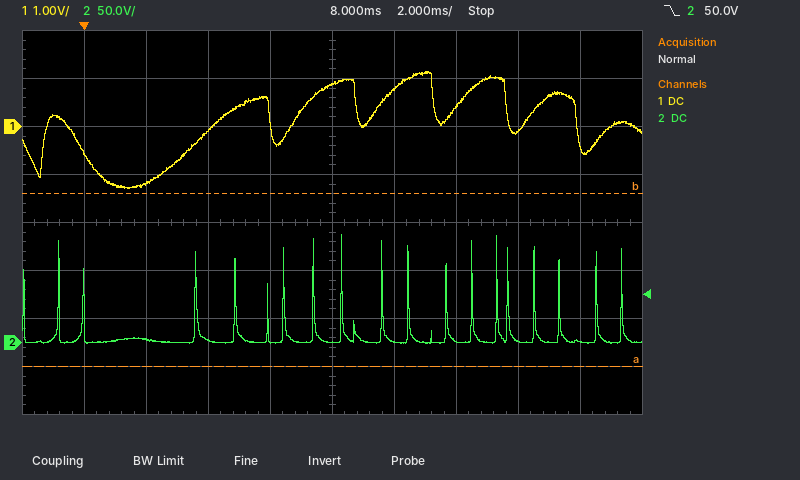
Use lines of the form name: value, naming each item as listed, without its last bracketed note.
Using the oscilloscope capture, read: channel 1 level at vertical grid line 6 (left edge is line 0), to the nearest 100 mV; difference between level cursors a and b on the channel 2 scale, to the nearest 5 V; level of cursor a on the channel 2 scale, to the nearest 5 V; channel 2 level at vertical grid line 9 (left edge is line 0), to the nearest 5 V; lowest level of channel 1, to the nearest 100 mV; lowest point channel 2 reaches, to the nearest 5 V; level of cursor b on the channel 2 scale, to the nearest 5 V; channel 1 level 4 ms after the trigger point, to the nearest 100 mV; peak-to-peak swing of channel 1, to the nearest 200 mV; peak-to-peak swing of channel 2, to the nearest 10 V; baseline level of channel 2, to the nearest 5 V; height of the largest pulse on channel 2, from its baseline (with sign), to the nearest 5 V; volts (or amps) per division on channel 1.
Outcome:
channel 1 level at vertical grid line 6 (left edge is line 0), to the nearest 100 mV: 800 mV
difference between level cursors a and b on the channel 2 scale, to the nearest 5 V: 180 V
level of cursor a on the channel 2 scale, to the nearest 5 V: -25 V
channel 2 level at vertical grid line 9 (left edge is line 0), to the nearest 5 V: 0 V
lowest level of channel 1, to the nearest 100 mV: -1.3 V
lowest point channel 2 reaches, to the nearest 5 V: 0 V
level of cursor b on the channel 2 scale, to the nearest 5 V: 155 V
channel 1 level 4 ms after the trigger point, to the nearest 100 mV: -100 mV
peak-to-peak swing of channel 1, to the nearest 200 mV: 2.4 V
peak-to-peak swing of channel 2, to the nearest 10 V: 110 V
baseline level of channel 2, to the nearest 5 V: 0 V
height of the largest pulse on channel 2, from its baseline (with sign), to the nearest 5 V: +110 V
volts (or amps) per division on channel 1: 1 V
